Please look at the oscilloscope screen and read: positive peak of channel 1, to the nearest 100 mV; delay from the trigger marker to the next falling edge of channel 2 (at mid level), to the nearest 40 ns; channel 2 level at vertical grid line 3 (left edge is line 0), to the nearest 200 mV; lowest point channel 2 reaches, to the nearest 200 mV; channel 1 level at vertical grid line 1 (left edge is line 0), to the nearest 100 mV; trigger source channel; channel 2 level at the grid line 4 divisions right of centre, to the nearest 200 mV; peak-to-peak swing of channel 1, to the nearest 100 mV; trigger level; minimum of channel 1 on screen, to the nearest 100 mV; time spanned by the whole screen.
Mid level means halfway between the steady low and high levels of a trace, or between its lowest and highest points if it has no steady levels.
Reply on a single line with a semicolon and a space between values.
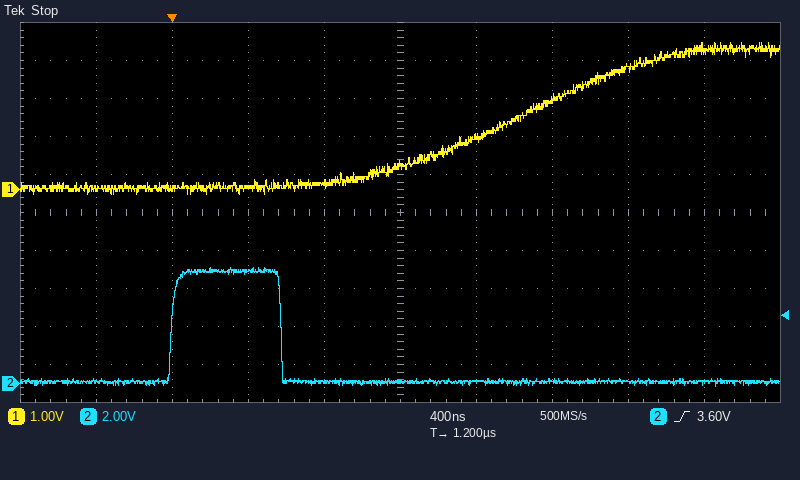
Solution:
3.9 V; 560 ns; 5.8 V; -200 mV; 0.0 V; channel 2; 0.0 V; 4.0 V; 3.60 V; -100 mV; 4 µs
